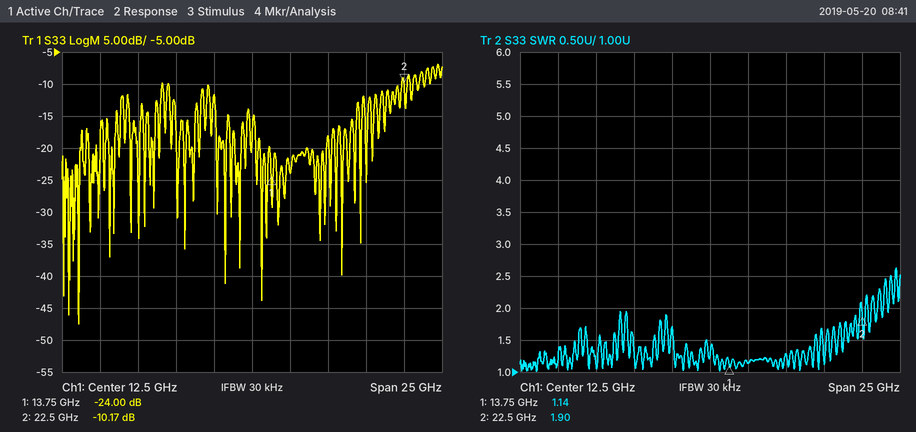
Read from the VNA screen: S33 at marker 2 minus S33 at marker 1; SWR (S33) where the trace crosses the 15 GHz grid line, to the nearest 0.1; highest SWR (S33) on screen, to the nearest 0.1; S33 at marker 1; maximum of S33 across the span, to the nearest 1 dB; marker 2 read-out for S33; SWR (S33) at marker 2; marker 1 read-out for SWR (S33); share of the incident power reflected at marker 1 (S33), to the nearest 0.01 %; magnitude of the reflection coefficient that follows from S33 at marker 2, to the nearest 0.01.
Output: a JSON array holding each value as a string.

["13.83 dB", "1.1", "2.6", "-24.00 dB", "-7 dB", "-10.17 dB", "1.90", "1.14", "0.40 %", "0.31"]
